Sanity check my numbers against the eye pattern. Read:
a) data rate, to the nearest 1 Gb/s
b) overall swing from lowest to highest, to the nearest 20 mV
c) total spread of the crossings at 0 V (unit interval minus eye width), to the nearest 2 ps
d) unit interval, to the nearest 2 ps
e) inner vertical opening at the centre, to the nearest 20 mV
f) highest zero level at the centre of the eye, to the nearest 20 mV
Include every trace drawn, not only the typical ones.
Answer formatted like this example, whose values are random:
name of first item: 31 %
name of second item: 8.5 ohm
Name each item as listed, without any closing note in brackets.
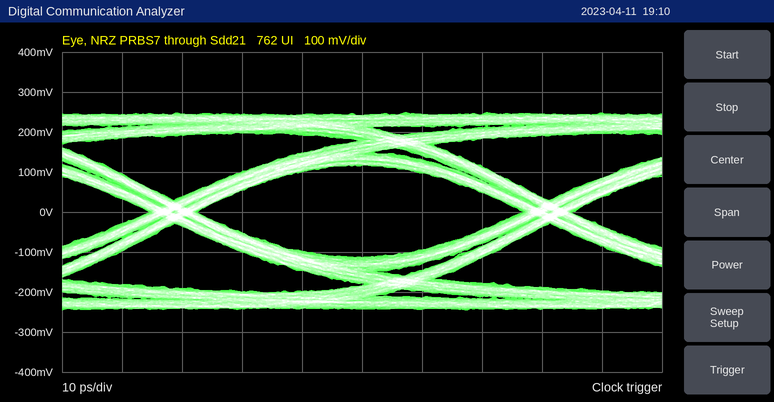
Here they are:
data rate, to the nearest 1 Gb/s: 16 Gb/s
overall swing from lowest to highest, to the nearest 20 mV: 500 mV
total spread of the crossings at 0 V (unit interval minus eye width), to the nearest 2 ps: 8 ps
unit interval, to the nearest 2 ps: 62 ps
inner vertical opening at the centre, to the nearest 20 mV: 240 mV
highest zero level at the centre of the eye, to the nearest 20 mV: -120 mV
